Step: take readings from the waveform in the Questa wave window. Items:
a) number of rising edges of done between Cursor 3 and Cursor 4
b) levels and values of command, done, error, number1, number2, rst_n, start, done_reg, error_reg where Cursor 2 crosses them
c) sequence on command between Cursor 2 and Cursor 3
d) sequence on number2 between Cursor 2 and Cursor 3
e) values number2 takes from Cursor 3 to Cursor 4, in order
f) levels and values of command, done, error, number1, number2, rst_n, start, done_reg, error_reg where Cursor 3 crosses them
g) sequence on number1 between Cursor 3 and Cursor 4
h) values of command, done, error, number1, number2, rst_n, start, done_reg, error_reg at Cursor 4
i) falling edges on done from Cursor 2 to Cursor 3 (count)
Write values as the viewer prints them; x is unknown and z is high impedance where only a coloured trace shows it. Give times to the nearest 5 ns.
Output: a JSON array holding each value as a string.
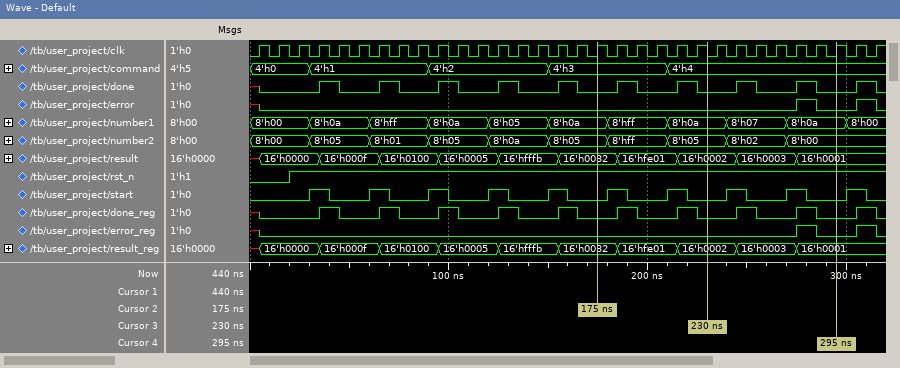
["2", "command=4'h3, done=0, error=0, number1=8'h0a, number2=8'h05, rst_n=1, start=0, done_reg=0, error_reg=0", "4'h3, 4'h4", "8'h05, 8'hff, 8'h05", "8'h05, 8'h02, 8'h00", "command=4'h4, done=0, error=0, number1=8'h0a, number2=8'h05, rst_n=1, start=0, done_reg=0, error_reg=0", "8'h0a, 8'h07, 8'h0a", "command=4'h4, done=0, error=0, number1=8'h0a, number2=8'h00, rst_n=1, start=0, done_reg=0, error_reg=0", "2"]
